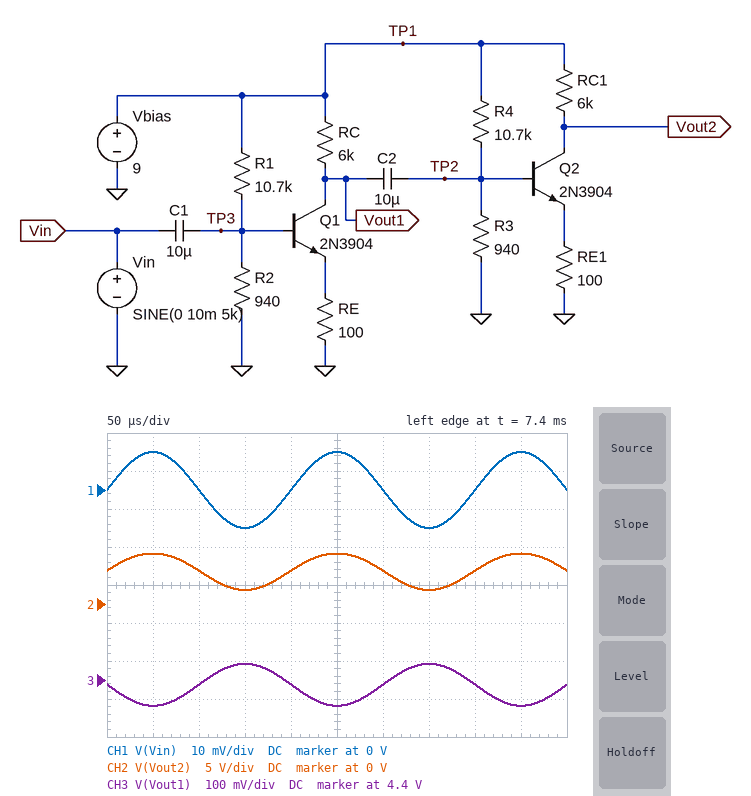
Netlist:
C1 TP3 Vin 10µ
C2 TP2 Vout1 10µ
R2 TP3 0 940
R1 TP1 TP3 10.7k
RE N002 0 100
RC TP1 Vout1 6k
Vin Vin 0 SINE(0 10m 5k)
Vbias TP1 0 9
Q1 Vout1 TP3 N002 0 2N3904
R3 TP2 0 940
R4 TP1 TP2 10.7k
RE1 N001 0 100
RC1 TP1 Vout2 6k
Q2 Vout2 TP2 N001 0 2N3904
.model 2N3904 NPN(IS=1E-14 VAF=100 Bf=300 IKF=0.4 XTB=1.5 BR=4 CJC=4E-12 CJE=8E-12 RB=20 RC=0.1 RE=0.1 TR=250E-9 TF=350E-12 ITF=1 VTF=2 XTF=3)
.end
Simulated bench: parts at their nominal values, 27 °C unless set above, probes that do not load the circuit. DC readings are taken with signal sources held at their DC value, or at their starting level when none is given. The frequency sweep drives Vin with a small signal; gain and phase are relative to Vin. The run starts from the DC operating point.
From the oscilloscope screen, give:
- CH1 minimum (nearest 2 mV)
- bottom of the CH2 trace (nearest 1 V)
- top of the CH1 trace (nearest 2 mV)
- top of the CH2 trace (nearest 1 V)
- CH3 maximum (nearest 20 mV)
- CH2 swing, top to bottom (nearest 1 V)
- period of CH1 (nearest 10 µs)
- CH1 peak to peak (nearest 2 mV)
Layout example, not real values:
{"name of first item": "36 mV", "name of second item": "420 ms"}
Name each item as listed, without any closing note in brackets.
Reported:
{"CH1 minimum": "-10 mV", "bottom of the CH2 trace": "2 V", "top of the CH1 trace": "10 mV", "top of the CH2 trace": "7 V", "CH3 maximum": "4.44 V", "CH2 swing, top to bottom": "5 V", "period of CH1": "200 µs", "CH1 peak to peak": "20 mV"}
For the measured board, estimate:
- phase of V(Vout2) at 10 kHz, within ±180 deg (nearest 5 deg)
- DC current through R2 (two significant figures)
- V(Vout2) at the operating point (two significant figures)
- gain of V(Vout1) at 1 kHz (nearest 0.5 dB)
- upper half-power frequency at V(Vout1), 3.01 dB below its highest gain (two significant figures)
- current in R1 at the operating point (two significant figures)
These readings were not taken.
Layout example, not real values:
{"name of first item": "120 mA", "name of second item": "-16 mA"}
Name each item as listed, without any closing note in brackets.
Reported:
{"phase of V(Vout2) at 10 kHz, within ±180 deg": "0 deg", "DC current through R2": "770 µA", "V(Vout2) at the operating point": "4.4 V", "gain of V(Vout1) at 1 kHz": "15.0 dB", "upper half-power frequency at V(Vout1), 3.01 dB below its highest gain": "1.7 MHz", "current in R1 at the operating point": "770 µA"}
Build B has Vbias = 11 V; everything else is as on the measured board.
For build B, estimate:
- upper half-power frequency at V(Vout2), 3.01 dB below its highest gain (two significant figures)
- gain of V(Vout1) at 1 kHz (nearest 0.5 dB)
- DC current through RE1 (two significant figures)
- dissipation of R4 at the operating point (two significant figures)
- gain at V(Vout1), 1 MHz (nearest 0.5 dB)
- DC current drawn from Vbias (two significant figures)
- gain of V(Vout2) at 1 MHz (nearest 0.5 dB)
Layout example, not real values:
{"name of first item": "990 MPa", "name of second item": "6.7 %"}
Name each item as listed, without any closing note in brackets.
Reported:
{"upper half-power frequency at V(Vout2), 3.01 dB below its highest gain": "180 kHz", "gain of V(Vout1) at 1 kHz": "-1.5 dB", "DC current through RE1": "1.8 mA", "dissipation of R4 at the operating point": "9.6 mW", "gain at V(Vout1), 1 MHz": "-3.5 dB", "DC current drawn from Vbias": "5.5 mA", "gain of V(Vout2) at 1 MHz": "-2.5 dB"}
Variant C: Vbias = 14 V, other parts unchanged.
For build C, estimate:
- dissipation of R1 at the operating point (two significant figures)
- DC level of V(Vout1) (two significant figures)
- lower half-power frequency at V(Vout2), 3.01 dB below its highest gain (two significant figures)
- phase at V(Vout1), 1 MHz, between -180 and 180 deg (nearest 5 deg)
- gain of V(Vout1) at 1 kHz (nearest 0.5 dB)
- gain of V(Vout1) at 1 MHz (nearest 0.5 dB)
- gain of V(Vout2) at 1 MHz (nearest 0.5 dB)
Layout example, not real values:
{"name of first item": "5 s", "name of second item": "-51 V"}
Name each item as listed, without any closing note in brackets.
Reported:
{"dissipation of R1 at the operating point": "16 mW", "DC level of V(Vout1)": "290 mV", "lower half-power frequency at V(Vout2), 3.01 dB below its highest gain": "420 kHz", "phase at V(Vout1), 1 MHz, between -180 and 180 deg": "15 deg", "gain of V(Vout1) at 1 kHz": "-25.0 dB", "gain of V(Vout1) at 1 MHz": "-3.0 dB", "gain of V(Vout2) at 1 MHz": "-5.0 dB"}
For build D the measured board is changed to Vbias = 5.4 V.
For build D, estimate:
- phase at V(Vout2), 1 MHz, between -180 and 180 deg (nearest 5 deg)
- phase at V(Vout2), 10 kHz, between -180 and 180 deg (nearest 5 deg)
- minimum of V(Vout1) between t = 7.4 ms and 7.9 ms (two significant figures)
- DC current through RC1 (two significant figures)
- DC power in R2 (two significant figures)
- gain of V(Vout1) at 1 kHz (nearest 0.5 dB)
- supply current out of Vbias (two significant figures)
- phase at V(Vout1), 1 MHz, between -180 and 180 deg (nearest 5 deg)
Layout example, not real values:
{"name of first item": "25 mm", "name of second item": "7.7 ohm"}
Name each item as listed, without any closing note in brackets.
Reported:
{"phase at V(Vout2), 1 MHz, between -180 and 180 deg": "-120 deg", "phase at V(Vout2), 10 kHz, between -180 and 180 deg": "0 deg", "minimum of V(Vout1) between t = 7.4 ms and 7.9 ms": "5.4 V", "DC current through RC1": "220 nA", "DC power in R2": "200 µW", "gain of V(Vout1) at 1 kHz": "-44.0 dB", "supply current out of Vbias": "930 µA", "phase at V(Vout1), 1 MHz, between -180 and 180 deg": "120 deg"}
